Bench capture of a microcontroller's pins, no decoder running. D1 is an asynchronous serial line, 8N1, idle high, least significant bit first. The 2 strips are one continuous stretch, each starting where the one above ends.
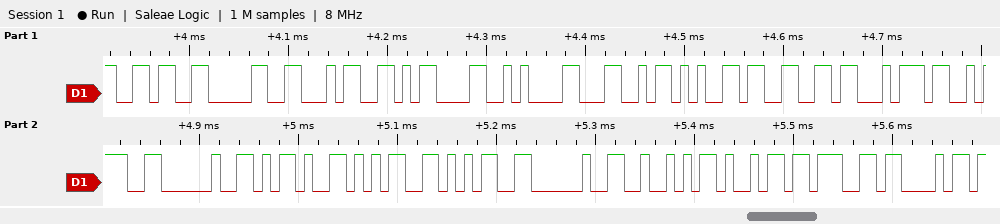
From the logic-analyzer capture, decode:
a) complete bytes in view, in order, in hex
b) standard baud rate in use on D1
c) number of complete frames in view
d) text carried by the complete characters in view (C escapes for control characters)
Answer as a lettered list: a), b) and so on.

a) 36 30 34 0D 0A 4C 65 66 74 3A 20 2D 35 35 20 52 69 67 68
b) 115200 baud
c) 19
d) "604\r\nLeft: -55 Righ"
